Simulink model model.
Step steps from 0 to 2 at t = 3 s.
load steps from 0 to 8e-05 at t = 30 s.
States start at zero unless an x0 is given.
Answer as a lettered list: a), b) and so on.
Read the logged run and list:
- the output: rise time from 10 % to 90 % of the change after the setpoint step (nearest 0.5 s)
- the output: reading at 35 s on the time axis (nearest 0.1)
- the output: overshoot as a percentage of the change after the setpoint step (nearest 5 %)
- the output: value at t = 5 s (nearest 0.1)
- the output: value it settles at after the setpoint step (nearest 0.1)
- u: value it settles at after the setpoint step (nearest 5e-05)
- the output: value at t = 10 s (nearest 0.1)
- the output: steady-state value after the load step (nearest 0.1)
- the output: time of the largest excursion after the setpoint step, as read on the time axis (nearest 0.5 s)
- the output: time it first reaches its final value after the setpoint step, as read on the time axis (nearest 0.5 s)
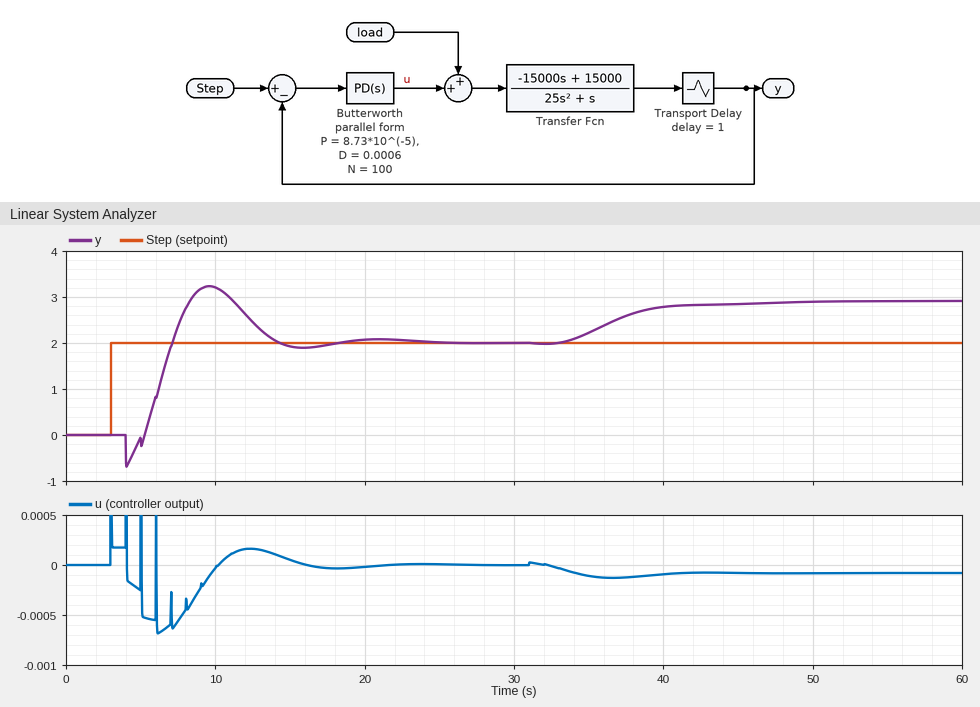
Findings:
a) 1.5 s
b) 2.2
c) 60 %
d) -0.1
e) 2.0
f) 0.00000
g) 3.2
h) 2.9
i) 9.5 s
j) 7.0 s
